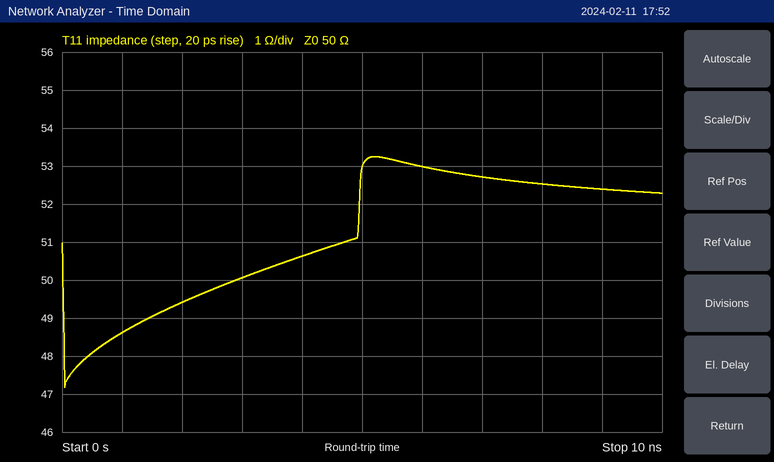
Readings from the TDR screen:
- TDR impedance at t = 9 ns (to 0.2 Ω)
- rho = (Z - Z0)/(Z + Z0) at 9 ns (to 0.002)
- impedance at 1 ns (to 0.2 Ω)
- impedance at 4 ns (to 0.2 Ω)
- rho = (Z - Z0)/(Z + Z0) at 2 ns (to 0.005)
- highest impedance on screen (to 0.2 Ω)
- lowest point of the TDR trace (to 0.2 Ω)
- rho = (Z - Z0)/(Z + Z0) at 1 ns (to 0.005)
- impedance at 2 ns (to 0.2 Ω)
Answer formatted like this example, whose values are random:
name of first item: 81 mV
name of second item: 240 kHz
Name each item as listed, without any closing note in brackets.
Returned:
TDR impedance at t = 9 ns: 52.4 Ω
rho = (Z - Z0)/(Z + Z0) at 9 ns: +0.024
impedance at 1 ns: 48.6 Ω
impedance at 4 ns: 50.6 Ω
rho = (Z - Z0)/(Z + Z0) at 2 ns: -0.005
highest impedance on screen: 53.2 Ω
lowest point of the TDR trace: 47.2 Ω
rho = (Z - Z0)/(Z + Z0) at 1 ns: -0.015
impedance at 2 ns: 49.4 Ω
